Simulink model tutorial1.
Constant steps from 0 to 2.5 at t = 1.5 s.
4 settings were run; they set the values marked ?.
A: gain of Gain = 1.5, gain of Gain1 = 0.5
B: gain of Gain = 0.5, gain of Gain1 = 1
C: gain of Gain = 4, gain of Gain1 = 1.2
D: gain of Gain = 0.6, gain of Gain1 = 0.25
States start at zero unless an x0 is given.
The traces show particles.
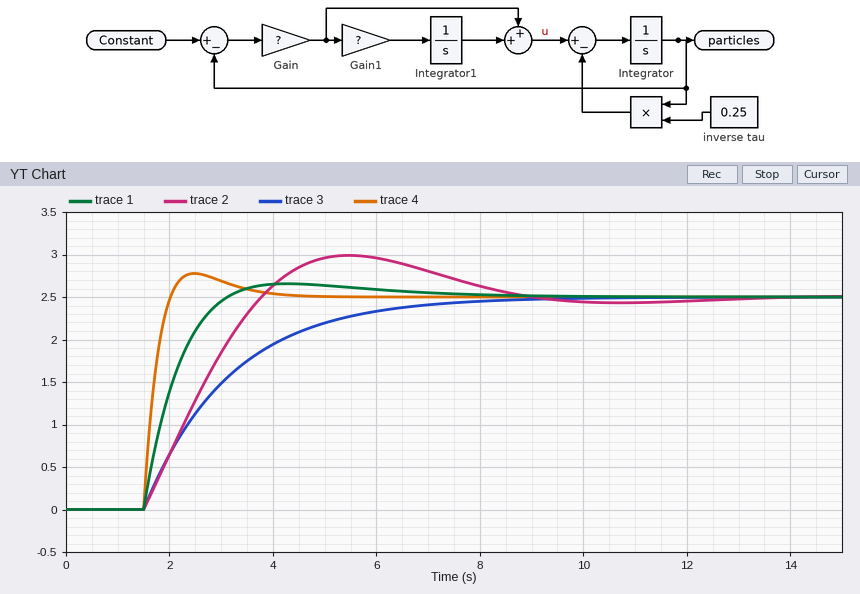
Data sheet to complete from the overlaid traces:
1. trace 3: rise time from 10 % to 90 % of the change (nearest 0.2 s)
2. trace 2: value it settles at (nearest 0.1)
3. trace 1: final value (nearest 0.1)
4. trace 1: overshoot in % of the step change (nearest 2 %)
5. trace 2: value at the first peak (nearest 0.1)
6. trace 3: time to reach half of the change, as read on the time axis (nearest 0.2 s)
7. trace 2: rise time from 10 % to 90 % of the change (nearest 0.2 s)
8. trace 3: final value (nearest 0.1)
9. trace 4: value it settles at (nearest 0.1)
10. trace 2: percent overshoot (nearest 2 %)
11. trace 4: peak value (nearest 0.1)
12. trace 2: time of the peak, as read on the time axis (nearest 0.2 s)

3.6 s
2.5
2.5
6 %
3.0
2.6 s
1.8 s
2.5
2.5
20 %
2.8
5.4 s
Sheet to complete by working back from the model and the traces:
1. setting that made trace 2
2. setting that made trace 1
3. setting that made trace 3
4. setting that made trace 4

B
A
D
C
